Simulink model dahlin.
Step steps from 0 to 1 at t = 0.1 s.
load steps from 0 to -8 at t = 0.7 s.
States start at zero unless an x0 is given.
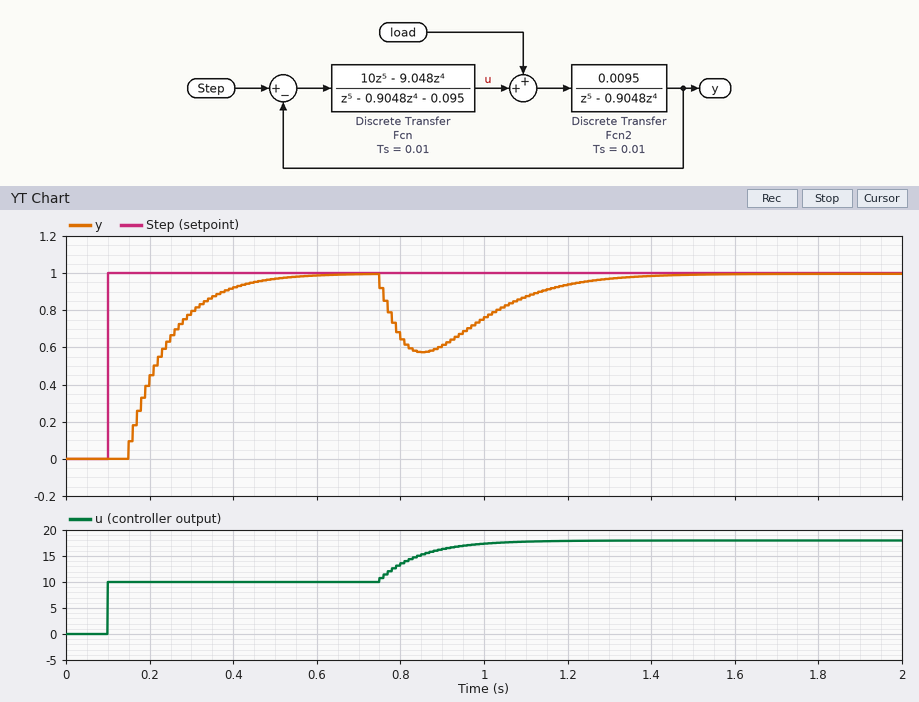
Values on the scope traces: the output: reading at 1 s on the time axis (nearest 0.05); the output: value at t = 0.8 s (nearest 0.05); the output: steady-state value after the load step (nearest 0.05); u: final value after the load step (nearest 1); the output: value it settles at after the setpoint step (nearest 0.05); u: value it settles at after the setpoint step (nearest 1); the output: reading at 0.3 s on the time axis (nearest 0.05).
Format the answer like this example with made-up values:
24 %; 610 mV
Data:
0.75; 0.65; 1.00; 18; 1.00; 10; 0.80
